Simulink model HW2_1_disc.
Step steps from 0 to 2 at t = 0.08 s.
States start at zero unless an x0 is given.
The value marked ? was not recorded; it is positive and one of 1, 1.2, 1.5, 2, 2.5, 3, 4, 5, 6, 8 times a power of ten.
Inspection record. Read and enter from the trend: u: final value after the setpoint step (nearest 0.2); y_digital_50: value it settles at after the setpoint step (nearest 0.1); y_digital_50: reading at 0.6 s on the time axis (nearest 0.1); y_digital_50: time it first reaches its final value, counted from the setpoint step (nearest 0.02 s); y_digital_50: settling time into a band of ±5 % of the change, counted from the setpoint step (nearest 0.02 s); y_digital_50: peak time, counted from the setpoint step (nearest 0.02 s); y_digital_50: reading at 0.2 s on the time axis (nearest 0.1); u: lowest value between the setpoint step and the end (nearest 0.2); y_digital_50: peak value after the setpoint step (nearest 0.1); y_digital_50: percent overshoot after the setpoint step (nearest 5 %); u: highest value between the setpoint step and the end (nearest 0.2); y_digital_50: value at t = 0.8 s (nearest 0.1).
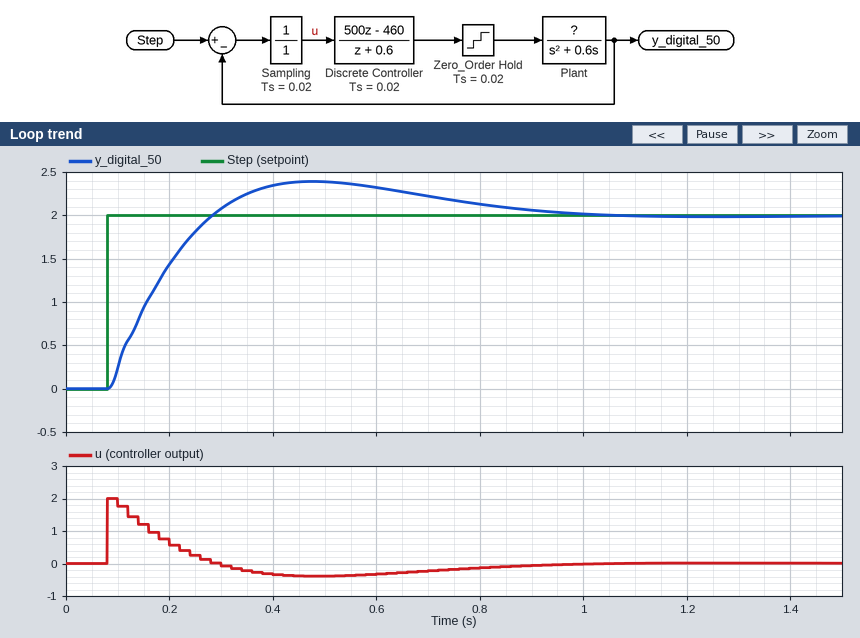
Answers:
0.0
2.0
2.3
0.20 s
0.76 s
0.40 s
1.4
-0.4
2.4
20 %
2.0
2.1
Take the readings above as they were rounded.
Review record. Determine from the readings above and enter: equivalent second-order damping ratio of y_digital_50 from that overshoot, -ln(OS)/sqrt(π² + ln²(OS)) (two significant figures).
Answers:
0.46
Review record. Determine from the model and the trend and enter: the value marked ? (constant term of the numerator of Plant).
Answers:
1.2
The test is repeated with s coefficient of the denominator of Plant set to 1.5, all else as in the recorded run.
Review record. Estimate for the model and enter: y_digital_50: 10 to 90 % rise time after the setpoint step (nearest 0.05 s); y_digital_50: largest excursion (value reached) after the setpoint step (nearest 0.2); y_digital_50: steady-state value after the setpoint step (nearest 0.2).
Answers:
0.15 s
2.2
2.0
